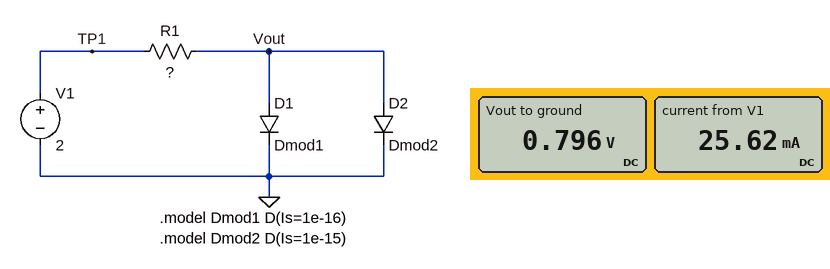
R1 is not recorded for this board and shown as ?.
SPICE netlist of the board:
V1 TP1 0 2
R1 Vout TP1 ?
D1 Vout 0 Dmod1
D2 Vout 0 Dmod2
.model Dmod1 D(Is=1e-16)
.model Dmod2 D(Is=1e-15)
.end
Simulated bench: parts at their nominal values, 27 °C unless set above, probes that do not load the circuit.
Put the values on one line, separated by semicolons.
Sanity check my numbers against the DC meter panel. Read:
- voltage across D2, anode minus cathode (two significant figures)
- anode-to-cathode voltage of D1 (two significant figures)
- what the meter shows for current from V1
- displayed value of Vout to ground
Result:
800 mV; 800 mV; 25.62 mA; 0.796 V
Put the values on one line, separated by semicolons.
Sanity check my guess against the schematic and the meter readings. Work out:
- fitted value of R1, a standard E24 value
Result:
47 Ω
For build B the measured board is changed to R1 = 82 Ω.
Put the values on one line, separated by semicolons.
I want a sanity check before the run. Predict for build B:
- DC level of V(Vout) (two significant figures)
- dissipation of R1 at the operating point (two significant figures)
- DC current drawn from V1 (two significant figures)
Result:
780 mV; 18 mW; 15 mA
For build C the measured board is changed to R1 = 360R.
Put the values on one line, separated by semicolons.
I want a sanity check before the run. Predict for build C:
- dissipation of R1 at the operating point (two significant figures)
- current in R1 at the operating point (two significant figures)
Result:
4.4 mW; 3.5 mA
